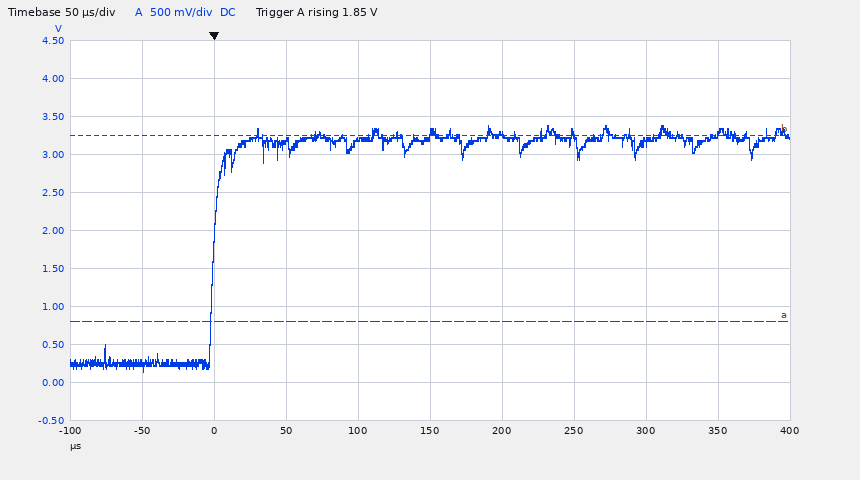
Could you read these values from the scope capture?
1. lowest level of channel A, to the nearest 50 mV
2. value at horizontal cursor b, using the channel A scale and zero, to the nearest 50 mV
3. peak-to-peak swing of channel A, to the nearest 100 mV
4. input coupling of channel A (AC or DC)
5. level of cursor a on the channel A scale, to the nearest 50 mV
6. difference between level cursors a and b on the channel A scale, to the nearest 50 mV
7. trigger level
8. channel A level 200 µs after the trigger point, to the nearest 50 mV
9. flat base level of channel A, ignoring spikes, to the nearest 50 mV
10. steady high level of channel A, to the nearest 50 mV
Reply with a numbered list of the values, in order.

1. 150 mV
2. 3.25 V
3. 3.20 V
4. DC
5. 800 mV
6. 2.45 V
7. 1.85 V
8. 3.25 V
9. 250 mV
10. 3.20 V
